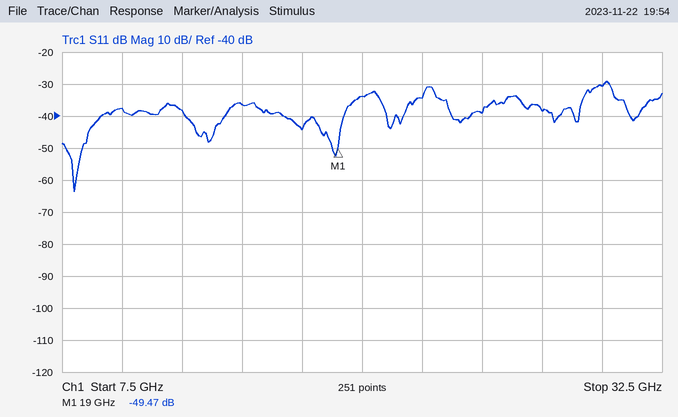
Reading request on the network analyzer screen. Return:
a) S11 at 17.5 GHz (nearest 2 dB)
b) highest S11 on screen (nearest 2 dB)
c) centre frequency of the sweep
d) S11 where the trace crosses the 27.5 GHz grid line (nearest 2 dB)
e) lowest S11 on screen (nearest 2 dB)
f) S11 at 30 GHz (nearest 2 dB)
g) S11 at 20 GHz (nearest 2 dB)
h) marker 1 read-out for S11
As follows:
-44 dB
-30 dB
20 GHz
-38 dB
-64 dB
-30 dB
-34 dB
-49.47 dB
